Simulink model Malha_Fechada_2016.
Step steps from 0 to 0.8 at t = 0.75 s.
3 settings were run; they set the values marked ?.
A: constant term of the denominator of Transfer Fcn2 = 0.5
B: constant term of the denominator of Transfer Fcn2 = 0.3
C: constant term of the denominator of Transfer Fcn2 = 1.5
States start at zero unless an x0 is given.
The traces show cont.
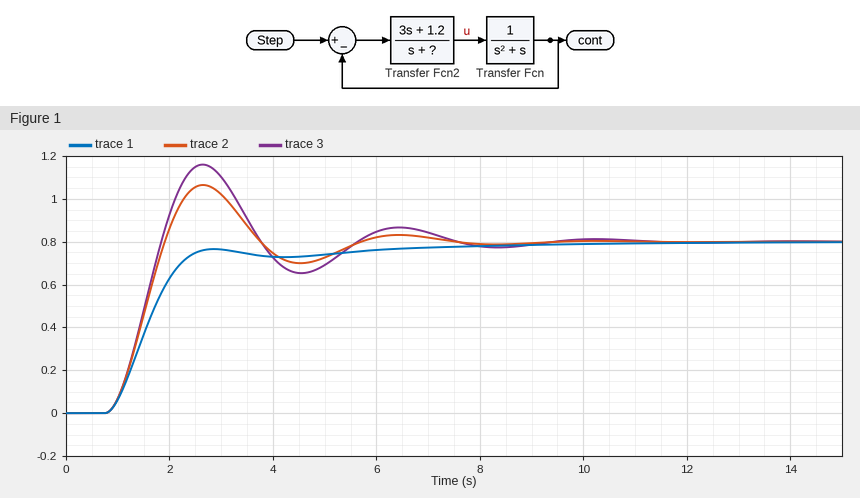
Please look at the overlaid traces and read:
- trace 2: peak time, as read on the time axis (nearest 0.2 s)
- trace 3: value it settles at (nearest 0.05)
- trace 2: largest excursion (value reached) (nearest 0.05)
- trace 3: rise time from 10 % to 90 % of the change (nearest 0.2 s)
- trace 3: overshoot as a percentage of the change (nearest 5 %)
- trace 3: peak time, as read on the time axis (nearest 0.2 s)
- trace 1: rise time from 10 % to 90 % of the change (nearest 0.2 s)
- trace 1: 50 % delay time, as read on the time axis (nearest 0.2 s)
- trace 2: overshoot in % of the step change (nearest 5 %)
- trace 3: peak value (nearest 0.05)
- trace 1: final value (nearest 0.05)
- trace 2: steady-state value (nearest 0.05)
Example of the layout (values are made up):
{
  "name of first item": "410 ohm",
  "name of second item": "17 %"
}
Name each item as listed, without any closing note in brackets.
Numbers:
{
  "trace 2: peak time, as read on the time axis": "2.6 s",
  "trace 3: value it settles at": "0.80",
  "trace 2: largest excursion (value reached)": "1.05",
  "trace 3: rise time from 10 % to 90 % of the change": "0.8 s",
  "trace 3: overshoot as a percentage of the change": "45 %",
  "trace 3: peak time, as read on the time axis": "2.6 s",
  "trace 1: rise time from 10 % to 90 % of the change": "1.2 s",
  "trace 1: 50 % delay time, as read on the time axis": "1.6 s",
  "trace 2: overshoot in % of the step change": "35 %",
  "trace 3: peak value": "1.15",
  "trace 1: final value": "0.80",
  "trace 2: steady-state value": "0.80"
}
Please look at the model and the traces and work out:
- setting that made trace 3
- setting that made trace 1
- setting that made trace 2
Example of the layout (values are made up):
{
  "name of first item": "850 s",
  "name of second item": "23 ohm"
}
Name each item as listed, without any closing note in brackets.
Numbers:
{
  "setting that made trace 3": "B",
  "setting that made trace 1": "C",
  "setting that made trace 2": "A"
}
